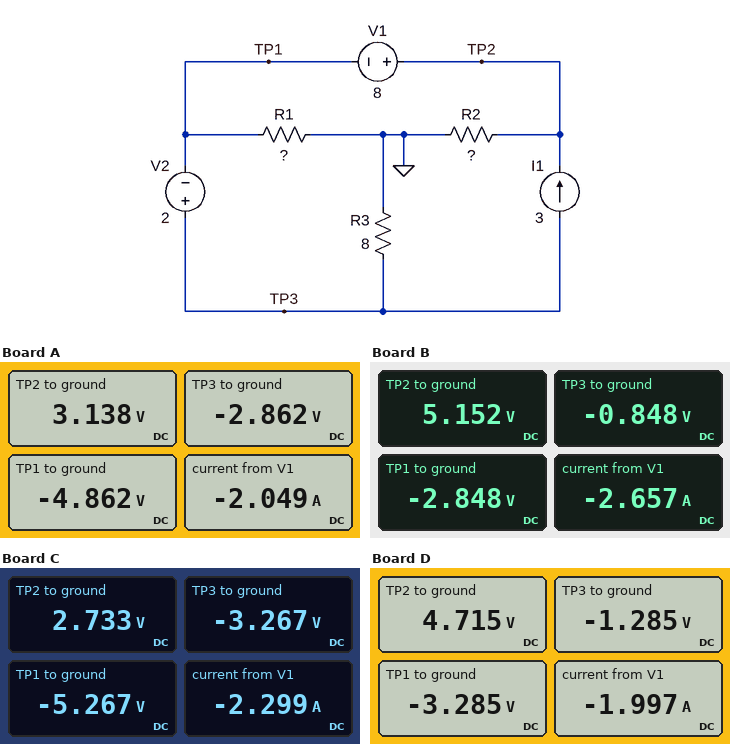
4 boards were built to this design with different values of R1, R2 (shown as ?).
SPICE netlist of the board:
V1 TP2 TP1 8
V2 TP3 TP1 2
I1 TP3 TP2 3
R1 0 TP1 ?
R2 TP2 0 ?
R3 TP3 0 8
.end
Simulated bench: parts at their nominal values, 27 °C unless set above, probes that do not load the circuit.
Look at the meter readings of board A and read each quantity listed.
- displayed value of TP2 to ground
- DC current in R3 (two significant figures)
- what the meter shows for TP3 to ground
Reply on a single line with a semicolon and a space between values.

3.138 V; 360 mA; -2.862 V
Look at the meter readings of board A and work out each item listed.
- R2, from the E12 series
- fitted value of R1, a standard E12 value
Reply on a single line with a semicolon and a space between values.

3.3 Ω; 8.2 Ω
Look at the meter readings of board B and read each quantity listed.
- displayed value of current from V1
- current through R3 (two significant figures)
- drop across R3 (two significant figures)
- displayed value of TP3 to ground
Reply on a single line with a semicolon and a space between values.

-2.657 A; 110 mA; 850 mV; -0.848 V
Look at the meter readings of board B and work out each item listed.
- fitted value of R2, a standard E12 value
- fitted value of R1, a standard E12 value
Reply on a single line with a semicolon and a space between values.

15 Ω; 12 Ω
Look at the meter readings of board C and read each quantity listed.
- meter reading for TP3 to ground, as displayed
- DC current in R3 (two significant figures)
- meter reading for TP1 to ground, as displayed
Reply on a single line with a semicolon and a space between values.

-3.267 V; 410 mA; -5.267 V
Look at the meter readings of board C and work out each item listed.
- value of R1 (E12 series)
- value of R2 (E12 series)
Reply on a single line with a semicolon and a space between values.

18 Ω; 3.9 Ω
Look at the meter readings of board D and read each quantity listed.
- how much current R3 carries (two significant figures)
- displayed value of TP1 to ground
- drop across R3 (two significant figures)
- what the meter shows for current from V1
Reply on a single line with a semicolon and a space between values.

160 mA; -3.285 V; 1.3 V; -1.997 A
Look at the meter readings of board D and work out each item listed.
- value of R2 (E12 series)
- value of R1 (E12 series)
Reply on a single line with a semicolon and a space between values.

4.7 Ω; 3.9 Ω
